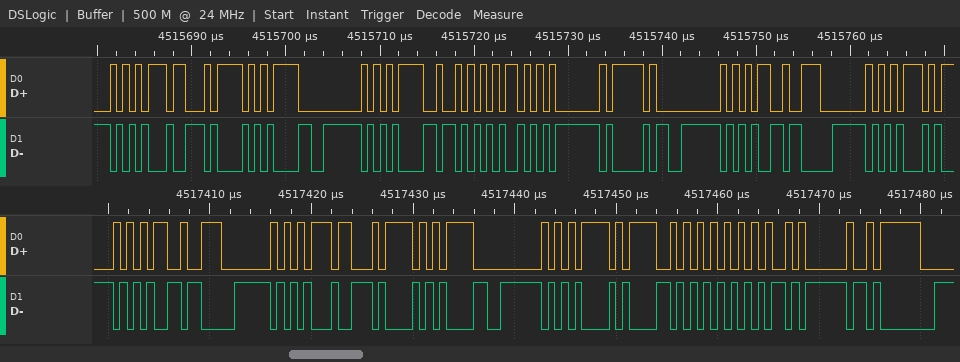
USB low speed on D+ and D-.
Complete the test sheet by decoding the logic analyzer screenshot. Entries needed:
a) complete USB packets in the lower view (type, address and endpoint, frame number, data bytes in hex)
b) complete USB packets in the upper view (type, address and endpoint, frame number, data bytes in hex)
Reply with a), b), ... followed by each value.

a) ACK, IN ADDR 28 EP 0, DATA0 [ 05 00 08 ]
b) IN ADDR 28 EP 0, DATA1 [ 00 01 ], ACK
